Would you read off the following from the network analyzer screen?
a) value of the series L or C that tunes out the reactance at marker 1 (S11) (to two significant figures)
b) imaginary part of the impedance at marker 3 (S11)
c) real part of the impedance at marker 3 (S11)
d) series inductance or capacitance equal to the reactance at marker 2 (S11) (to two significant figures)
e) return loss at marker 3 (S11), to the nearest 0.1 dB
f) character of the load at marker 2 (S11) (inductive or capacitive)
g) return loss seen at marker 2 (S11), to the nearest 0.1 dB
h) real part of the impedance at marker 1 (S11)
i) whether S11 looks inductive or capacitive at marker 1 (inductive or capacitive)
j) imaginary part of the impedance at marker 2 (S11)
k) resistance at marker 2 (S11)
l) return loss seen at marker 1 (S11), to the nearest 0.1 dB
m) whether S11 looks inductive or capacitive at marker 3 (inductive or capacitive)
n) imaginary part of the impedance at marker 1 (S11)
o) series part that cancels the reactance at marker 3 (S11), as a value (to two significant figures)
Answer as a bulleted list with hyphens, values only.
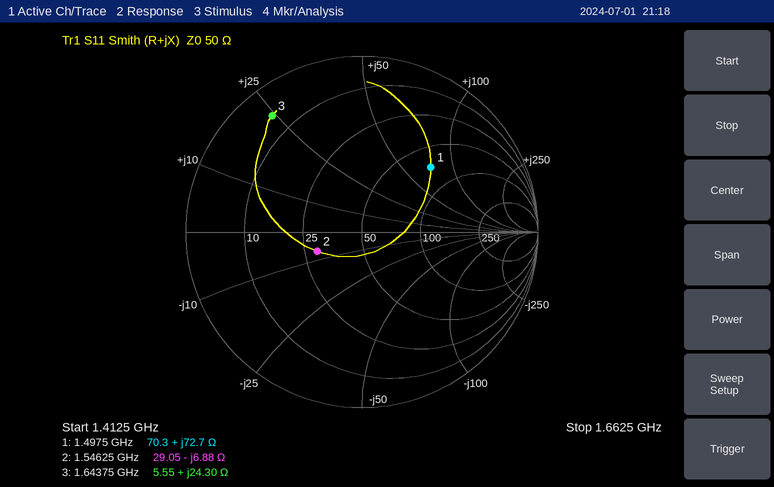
- 1.5 pF
- +24.30 Ω
- 5.55 Ω
- 15 pF
- 1.6 dB
- capacitive
- 11.1 dB
- 70.3 Ω
- inductive
- -6.88 Ω
- 29.05 Ω
- 5.4 dB
- inductive
- +72.7 Ω
- 4.0 pF
